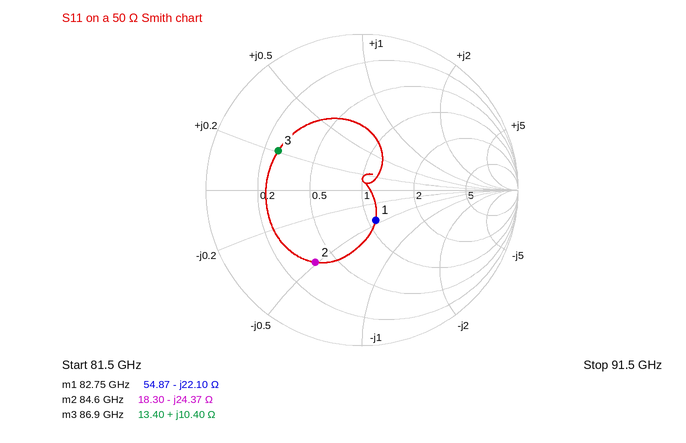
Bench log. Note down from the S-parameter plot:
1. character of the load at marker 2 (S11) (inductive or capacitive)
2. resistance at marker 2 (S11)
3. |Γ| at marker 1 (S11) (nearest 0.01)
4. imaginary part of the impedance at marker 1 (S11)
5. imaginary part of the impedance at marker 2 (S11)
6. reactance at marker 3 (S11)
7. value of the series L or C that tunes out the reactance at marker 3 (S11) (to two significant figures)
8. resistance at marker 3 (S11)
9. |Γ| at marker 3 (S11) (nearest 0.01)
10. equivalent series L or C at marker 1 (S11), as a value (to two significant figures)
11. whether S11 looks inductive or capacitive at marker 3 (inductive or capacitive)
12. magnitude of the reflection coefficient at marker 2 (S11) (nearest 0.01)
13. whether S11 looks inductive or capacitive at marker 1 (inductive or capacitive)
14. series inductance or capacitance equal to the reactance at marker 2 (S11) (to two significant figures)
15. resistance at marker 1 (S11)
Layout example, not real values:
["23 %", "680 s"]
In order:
["capacitive", "18.30 Ω", "0.21", "-22.10 Ω", "-24.37 Ω", "+10.40 Ω", "180 fF", "13.40 Ω", "0.59", "87 fF", "inductive", "0.55", "capacitive", "77 fF", "54.87 Ω"]
